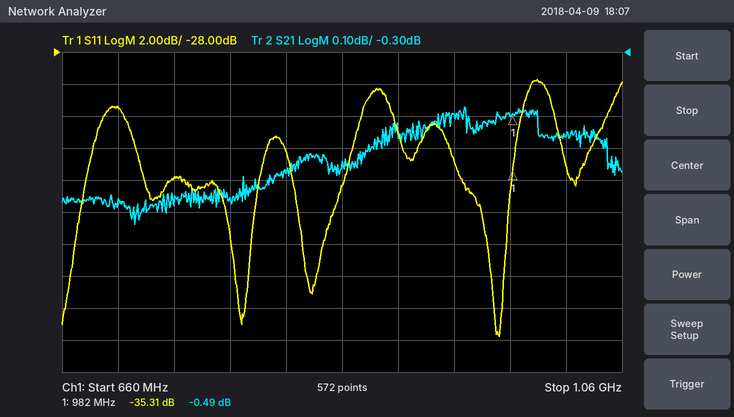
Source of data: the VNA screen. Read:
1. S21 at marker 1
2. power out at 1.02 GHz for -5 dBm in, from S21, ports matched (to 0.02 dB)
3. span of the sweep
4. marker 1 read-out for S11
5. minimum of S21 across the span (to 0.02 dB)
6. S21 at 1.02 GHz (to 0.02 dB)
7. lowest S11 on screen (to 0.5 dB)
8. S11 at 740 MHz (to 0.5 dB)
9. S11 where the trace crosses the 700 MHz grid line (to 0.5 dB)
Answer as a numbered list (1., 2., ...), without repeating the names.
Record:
1. -0.49 dB
2. -5.56 dBm
3. 400 MHz
4. -35.31 dB
5. -0.84 dB
6. -0.56 dB
7. -46.0 dB
8. -36.0 dB
9. -31.5 dB
